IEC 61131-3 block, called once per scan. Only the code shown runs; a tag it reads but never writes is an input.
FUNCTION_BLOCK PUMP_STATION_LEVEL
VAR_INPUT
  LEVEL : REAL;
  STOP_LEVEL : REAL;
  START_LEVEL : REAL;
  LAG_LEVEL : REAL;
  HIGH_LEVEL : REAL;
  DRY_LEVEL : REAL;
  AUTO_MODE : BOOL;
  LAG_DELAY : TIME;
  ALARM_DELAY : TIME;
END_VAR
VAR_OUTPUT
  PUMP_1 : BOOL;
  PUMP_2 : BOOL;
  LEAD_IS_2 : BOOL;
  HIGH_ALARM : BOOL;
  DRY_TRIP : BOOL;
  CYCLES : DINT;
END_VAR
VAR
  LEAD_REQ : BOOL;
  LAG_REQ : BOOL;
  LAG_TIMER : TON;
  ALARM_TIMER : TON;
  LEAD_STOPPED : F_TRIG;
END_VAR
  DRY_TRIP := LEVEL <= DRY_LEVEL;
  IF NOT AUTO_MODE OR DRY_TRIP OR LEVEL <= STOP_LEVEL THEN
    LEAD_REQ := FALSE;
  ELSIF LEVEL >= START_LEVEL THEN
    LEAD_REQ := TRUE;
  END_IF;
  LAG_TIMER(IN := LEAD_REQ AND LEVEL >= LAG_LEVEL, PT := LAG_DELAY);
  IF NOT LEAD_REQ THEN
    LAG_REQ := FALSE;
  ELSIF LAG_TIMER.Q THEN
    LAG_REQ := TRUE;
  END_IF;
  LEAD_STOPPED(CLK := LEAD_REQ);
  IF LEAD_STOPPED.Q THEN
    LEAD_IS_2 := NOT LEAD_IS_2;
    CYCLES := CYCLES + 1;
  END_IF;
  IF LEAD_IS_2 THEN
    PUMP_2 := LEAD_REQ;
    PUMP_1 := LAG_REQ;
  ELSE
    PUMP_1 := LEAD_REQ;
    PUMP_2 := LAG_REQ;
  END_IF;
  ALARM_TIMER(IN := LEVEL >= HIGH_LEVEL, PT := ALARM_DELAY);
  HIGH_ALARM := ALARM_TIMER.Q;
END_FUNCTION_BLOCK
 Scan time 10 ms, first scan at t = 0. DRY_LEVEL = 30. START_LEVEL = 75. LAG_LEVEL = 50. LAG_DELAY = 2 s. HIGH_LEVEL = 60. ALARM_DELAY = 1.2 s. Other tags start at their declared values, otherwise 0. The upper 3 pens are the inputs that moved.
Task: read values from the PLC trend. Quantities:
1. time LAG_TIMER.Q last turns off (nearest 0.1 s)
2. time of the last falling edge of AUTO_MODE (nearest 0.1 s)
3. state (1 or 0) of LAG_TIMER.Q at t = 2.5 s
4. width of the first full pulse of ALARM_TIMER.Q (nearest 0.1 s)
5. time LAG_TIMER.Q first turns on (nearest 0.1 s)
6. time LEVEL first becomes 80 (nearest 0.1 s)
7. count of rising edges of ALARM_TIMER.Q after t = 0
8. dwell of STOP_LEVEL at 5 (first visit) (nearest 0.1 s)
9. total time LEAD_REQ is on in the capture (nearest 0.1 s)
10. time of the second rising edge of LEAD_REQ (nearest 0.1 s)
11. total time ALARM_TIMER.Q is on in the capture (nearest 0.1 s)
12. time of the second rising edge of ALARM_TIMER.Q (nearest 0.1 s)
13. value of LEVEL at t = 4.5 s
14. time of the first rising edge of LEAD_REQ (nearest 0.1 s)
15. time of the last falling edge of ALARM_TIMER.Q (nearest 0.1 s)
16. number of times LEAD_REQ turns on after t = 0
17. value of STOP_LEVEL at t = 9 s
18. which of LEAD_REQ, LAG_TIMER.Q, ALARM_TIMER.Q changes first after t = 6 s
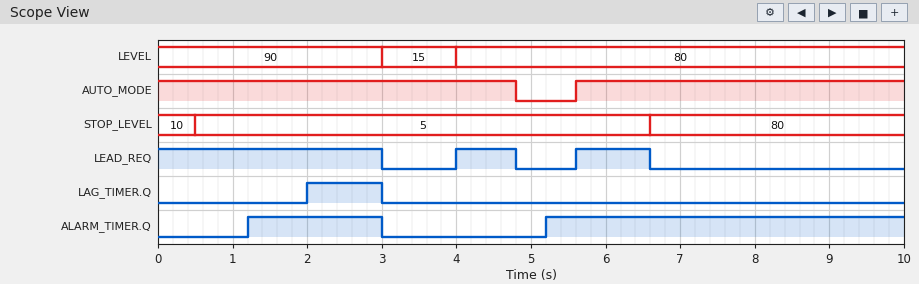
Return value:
3.0 s
4.8 s
1
1.8 s
2.0 s
4.0 s
2
6.1 s
4.8 s
5.6 s
6.6 s
5.2 s
80
4.0 s
3.0 s
2
80
LEAD_REQ
